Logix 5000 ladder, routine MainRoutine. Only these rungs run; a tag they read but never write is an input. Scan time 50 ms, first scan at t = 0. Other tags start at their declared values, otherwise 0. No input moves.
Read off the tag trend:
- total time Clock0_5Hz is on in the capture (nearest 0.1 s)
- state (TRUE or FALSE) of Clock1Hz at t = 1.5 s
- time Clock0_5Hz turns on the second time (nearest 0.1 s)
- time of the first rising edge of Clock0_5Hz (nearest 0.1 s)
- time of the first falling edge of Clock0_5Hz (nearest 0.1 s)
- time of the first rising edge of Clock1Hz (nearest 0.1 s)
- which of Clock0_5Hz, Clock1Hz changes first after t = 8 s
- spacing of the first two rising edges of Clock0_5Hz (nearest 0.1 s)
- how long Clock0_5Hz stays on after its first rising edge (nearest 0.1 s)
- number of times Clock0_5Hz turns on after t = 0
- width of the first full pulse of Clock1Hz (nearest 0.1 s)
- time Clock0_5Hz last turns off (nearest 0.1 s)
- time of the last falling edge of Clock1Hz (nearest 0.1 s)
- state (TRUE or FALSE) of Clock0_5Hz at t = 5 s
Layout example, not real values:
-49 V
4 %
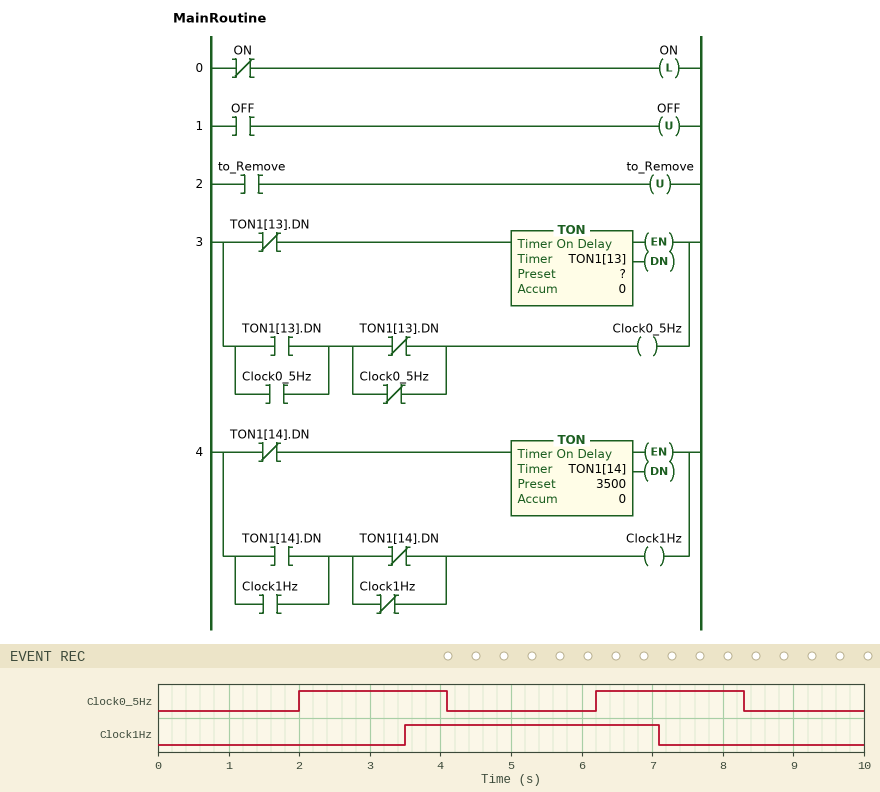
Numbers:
4.2 s
FALSE
6.2 s
2.0 s
4.1 s
3.5 s
Clock0_5Hz
4.2 s
2.1 s
2
3.6 s
8.3 s
7.1 s
FALSE
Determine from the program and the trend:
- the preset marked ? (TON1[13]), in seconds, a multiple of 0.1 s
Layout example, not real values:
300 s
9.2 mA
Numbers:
2.0 s
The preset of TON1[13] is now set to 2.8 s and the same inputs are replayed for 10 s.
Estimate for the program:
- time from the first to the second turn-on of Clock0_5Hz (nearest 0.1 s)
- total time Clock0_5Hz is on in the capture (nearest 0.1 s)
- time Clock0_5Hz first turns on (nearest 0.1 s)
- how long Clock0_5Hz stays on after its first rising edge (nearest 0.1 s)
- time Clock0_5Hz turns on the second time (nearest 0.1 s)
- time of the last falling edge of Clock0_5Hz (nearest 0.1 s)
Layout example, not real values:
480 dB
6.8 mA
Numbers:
5.8 s
4.3 s
2.8 s
2.9 s
8.6 s
5.7 s
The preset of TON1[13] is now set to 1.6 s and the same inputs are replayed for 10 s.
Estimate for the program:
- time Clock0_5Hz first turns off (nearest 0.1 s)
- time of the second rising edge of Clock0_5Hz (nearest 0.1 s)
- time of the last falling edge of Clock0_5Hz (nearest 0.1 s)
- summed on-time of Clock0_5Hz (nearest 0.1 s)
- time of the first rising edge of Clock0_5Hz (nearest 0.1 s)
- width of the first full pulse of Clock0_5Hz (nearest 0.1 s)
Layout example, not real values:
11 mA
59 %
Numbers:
3.3 s
5.0 s
6.7 s
5.0 s
1.6 s
1.7 s
